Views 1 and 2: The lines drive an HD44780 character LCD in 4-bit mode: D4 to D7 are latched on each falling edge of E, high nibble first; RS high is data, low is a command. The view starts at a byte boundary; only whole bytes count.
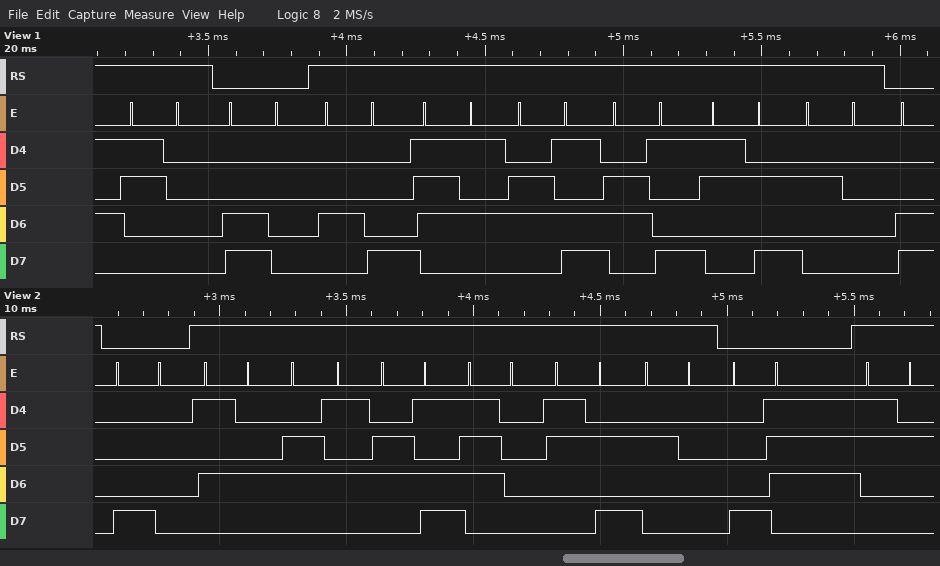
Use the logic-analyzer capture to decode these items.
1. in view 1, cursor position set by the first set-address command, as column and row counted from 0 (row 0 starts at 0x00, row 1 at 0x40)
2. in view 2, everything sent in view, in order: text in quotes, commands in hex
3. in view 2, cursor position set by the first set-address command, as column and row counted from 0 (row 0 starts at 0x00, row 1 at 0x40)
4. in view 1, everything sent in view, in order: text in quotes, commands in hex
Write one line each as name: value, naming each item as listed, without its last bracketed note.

in view 1, cursor position set by the first set-address command, as column and row counted from 0: column 0, row 1
in view 2, everything sent in view, in order: text in quotes, commands in hex: 0x80 "Temp: " 0x87 "2"
in view 2, cursor position set by the first set-address command, as column and row counted from 0: column 0, row 0
in view 1, everything sent in view, in order: text in quotes, commands in hex: "0" 0xC0 "Humi: "
